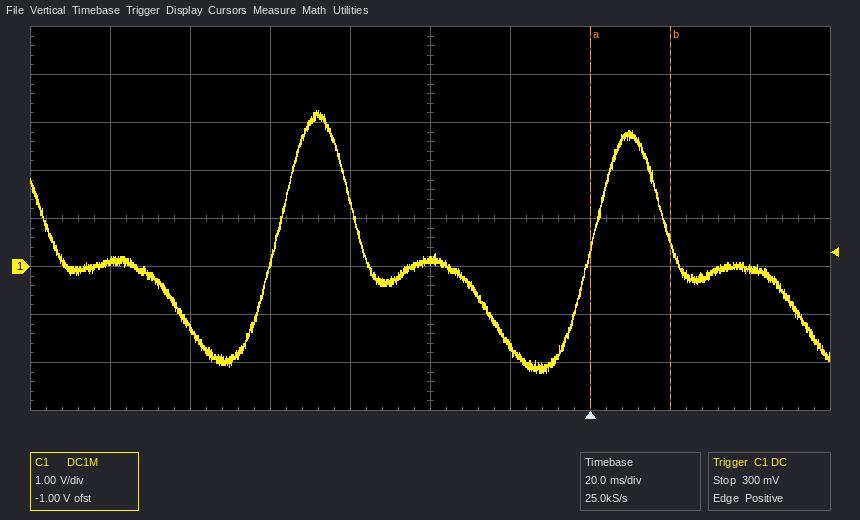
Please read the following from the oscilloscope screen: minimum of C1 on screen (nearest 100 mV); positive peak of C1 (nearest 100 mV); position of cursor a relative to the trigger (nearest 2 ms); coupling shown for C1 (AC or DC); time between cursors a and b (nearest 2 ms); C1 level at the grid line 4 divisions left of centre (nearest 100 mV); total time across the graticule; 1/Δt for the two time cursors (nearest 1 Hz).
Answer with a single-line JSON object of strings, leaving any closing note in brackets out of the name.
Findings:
{"minimum of C1 on screen": "-2.2 V", "positive peak of C1": "3.2 V", "position of cursor a relative to the trigger": "0 ms", "coupling shown for C1": "DC", "time between cursors a and b": "20 ms", "C1 level at the grid line 4 divisions left of centre": "100 mV", "total time across the graticule": "200 ms", "1/Δt for the two time cursors": "50 Hz"}
